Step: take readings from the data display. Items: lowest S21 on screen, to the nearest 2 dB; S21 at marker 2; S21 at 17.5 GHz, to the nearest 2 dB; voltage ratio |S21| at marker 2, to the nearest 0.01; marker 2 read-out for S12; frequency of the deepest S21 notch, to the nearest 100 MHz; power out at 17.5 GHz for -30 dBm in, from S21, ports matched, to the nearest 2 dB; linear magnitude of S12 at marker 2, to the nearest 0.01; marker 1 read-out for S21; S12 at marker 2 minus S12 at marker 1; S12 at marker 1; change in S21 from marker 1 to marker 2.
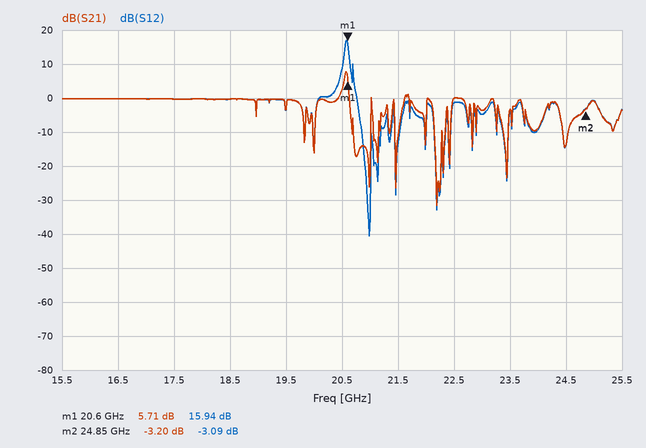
-32 dB
-3.20 dB
0 dB
0.69
-3.09 dB
22.2 GHz
-30 dBm
0.70
5.71 dB
-19.03 dB
15.94 dB
-8.91 dB
